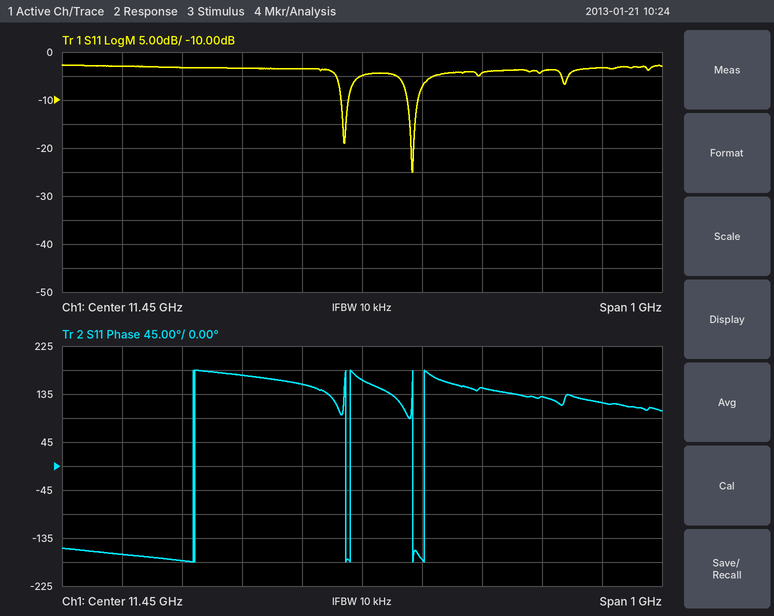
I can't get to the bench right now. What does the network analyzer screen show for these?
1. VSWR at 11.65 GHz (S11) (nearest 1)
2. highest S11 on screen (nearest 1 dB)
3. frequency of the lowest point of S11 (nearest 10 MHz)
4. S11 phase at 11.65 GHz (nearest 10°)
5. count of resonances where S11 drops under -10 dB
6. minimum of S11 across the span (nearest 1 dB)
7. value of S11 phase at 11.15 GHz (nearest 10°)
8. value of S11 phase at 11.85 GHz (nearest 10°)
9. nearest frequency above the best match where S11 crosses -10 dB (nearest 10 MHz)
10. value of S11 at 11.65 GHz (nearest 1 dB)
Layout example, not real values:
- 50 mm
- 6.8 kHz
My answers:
- 4
- -3 dB
- 11.53 GHz
- 150°
- 2
- -25 dB
- -180°
- 120°
- 11.54 GHz
- -4 dB
